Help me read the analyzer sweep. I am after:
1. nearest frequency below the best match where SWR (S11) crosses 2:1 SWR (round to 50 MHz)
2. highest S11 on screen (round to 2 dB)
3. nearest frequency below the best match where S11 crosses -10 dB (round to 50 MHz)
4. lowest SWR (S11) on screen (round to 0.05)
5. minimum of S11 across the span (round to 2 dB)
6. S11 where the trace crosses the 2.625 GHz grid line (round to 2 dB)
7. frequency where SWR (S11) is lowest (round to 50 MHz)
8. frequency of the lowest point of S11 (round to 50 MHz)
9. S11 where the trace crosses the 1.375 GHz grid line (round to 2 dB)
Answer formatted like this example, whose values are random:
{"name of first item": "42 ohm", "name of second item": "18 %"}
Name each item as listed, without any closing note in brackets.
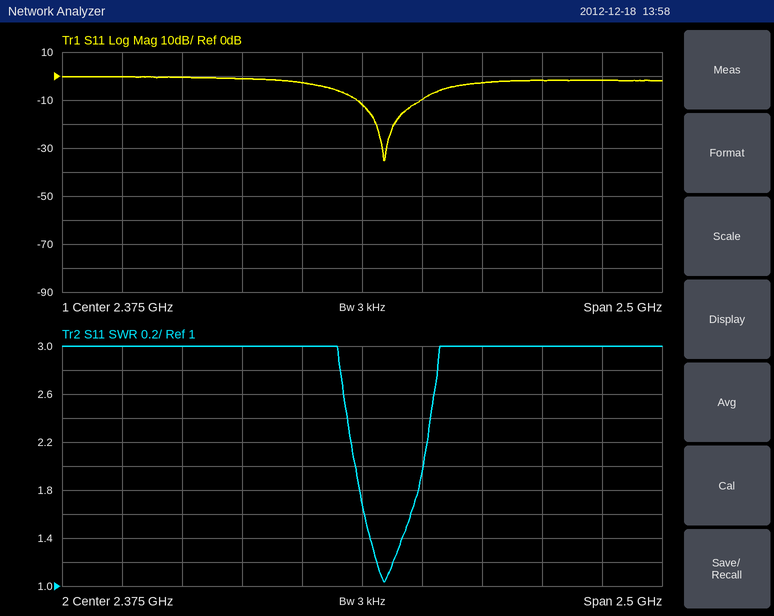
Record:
{"nearest frequency below the best match where SWR (S11) crosses 2:1 SWR": "2.35 GHz", "highest S11 on screen": "0 dB", "nearest frequency below the best match where S11 crosses -10 dB": "2.35 GHz", "lowest SWR (S11) on screen": "1.05", "minimum of S11 across the span": "-36 dB", "S11 where the trace crosses the 2.625 GHz grid line": "-10 dB", "frequency where SWR (S11) is lowest": "2.45 GHz", "frequency of the lowest point of S11": "2.45 GHz", "S11 where the trace crosses the 1.375 GHz grid line": "0 dB"}
